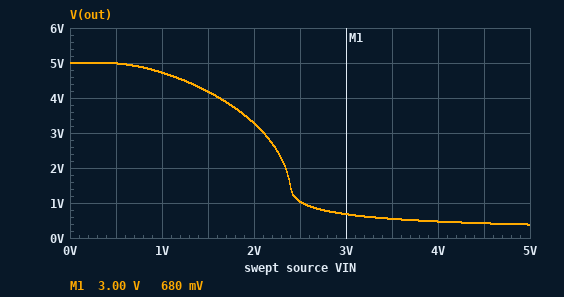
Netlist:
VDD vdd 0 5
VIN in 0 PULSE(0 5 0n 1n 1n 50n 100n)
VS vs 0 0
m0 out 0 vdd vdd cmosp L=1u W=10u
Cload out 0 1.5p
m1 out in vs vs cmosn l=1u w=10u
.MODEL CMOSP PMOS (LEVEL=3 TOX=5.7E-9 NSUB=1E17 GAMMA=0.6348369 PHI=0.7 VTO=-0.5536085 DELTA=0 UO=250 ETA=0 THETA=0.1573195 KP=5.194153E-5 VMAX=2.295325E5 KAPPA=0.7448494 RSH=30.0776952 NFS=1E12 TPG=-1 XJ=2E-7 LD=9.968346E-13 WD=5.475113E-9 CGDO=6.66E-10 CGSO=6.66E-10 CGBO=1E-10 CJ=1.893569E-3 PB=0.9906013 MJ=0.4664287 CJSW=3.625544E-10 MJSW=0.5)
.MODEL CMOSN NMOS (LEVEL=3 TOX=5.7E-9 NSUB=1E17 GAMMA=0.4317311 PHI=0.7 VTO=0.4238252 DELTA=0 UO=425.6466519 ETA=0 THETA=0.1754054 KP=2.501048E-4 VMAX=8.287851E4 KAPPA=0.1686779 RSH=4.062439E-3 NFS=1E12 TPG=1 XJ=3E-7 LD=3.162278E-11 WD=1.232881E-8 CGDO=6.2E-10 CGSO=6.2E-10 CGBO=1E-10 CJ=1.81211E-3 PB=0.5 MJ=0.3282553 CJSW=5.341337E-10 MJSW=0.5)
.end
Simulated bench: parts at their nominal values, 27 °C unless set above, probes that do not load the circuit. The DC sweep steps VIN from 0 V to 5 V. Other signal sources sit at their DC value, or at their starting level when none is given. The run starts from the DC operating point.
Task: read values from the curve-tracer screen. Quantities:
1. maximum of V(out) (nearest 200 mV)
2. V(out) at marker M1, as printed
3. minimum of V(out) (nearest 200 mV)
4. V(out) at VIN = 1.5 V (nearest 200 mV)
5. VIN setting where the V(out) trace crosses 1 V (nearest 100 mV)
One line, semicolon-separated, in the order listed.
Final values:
5.0 V; 680 mV; 400 mV; 4.2 V; 2.5 V
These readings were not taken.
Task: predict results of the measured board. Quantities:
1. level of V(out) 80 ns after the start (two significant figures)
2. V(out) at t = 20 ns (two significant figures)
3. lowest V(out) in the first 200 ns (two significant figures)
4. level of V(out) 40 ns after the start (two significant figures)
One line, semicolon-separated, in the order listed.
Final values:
5.0 V; 380 mV; 380 mV; 380 mV
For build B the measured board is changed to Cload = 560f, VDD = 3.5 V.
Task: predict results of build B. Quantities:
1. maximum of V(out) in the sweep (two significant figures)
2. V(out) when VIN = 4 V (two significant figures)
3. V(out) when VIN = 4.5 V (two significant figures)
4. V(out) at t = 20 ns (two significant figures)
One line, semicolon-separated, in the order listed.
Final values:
3.5 V; 230 mV; 210 mV; 190 mV
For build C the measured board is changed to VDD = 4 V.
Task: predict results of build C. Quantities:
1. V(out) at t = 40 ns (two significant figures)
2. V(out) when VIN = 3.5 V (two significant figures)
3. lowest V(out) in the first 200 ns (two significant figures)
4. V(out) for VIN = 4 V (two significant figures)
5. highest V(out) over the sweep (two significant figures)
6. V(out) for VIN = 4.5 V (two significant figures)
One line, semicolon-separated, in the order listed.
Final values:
250 mV; 340 mV; 240 mV; 300 mV; 4.0 V; 270 mV
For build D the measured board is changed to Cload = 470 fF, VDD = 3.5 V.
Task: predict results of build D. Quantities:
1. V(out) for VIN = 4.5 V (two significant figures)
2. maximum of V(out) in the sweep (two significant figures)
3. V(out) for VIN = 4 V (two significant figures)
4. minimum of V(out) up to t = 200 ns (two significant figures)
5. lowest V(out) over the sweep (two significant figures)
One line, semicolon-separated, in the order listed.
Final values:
210 mV; 3.5 V; 230 mV; 170 mV; 190 mV
